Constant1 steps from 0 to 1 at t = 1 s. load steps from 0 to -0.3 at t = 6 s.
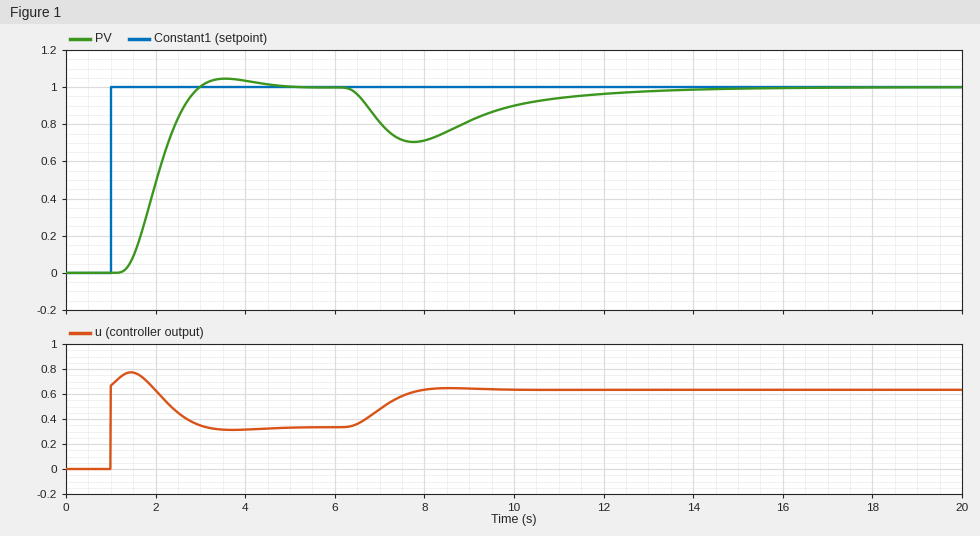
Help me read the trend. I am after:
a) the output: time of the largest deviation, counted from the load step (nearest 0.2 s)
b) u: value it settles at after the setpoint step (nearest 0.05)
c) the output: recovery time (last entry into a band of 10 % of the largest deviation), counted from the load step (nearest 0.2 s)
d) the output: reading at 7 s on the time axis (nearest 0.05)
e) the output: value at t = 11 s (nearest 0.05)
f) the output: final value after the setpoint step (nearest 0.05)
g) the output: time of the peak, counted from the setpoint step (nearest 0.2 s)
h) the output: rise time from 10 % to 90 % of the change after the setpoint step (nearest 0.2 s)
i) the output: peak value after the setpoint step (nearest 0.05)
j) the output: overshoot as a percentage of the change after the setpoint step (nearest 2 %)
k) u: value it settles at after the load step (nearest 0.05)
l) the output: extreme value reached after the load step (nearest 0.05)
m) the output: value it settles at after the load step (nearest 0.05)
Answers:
1.8 s
0.35
6.4 s
0.80
0.95
1.00
2.6 s
1.2 s
1.05
4 %
0.65
0.70
1.00
